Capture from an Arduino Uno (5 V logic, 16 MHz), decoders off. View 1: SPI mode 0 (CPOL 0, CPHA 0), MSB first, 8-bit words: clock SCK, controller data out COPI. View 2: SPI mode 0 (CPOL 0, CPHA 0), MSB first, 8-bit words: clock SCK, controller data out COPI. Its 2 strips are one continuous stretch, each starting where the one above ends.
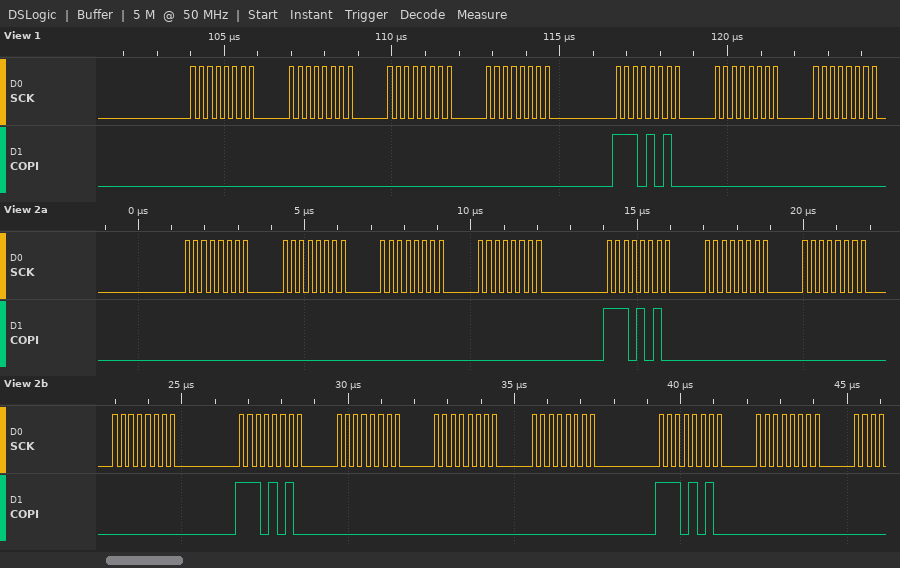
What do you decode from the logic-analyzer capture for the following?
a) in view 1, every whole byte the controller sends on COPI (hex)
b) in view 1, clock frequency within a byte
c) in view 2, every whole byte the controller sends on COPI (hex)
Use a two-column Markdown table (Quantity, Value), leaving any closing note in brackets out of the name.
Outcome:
| Quantity | Value |
|---|---|
| in view 1, every whole byte the controller sends on COPI | 00 00 00 00 EA 00 00 |
| in view 1, clock frequency within a byte | 4 MHz |
| in view 2, every whole byte the controller sends on COPI | 00 00 00 00 EA 00 00 00 EA 00 00 00 EA 00 |
